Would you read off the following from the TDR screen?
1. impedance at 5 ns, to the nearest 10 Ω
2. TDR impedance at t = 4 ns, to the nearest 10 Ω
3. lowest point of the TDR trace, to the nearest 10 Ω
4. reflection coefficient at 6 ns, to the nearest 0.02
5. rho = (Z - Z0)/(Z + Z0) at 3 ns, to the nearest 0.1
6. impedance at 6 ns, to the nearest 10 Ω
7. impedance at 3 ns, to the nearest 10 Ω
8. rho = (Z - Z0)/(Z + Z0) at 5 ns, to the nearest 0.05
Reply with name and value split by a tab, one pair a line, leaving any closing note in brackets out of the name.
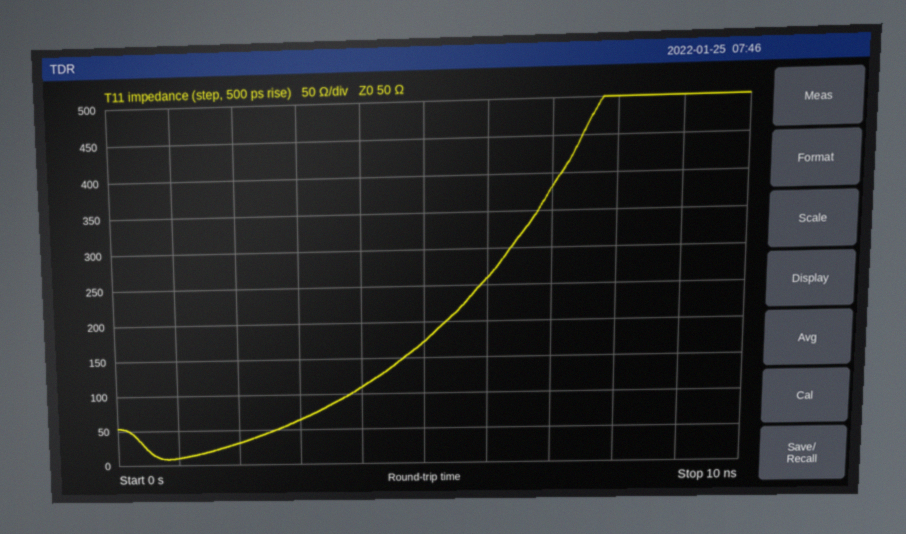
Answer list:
impedance at 5 ns, to the nearest 10 Ω	170 Ω
TDR impedance at t = 4 ns, to the nearest 10 Ω	110 Ω
lowest point of the TDR trace, to the nearest 10 Ω	10 Ω
reflection coefficient at 6 ns, to the nearest 0.02	+0.68
rho = (Z - Z0)/(Z + Z0) at 3 ns, to the nearest 0.1	+0.1
impedance at 6 ns, to the nearest 10 Ω	260 Ω
impedance at 3 ns, to the nearest 10 Ω	60 Ω
rho = (Z - Z0)/(Z + Z0) at 5 ns, to the nearest 0.05	+0.55
